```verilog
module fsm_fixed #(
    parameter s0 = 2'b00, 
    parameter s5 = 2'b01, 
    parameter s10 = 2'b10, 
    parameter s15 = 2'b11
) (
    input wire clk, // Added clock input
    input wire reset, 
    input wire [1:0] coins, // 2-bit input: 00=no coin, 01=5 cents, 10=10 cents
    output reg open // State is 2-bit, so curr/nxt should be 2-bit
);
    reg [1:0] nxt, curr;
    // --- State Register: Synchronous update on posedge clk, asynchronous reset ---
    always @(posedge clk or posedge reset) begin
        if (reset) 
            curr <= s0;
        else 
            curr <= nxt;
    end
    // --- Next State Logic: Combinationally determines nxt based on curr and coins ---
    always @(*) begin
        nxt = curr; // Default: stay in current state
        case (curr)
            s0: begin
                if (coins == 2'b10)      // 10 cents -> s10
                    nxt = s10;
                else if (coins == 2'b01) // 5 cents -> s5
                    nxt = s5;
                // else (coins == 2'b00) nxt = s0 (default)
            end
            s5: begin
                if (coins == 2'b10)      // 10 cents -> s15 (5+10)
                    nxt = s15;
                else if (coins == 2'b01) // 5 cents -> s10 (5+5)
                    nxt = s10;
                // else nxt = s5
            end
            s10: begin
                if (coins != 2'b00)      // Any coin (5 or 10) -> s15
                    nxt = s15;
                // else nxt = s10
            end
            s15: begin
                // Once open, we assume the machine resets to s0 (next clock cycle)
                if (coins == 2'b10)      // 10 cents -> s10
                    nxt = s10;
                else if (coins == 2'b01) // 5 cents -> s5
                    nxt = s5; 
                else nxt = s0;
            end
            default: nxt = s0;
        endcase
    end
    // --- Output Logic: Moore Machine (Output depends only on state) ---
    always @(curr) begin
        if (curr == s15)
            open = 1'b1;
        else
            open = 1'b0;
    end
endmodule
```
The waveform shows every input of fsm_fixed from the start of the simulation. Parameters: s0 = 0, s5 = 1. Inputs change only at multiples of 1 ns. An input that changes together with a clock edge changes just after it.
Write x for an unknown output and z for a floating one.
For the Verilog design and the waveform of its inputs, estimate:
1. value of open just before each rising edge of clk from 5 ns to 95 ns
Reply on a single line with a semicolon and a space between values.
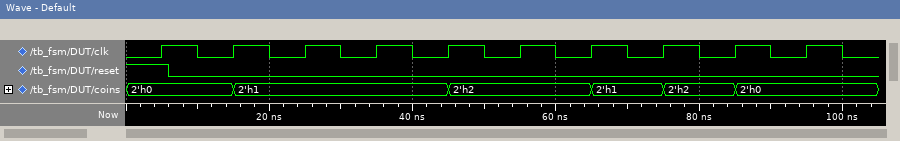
0 0 0 0 0 1 0 1 0 1
